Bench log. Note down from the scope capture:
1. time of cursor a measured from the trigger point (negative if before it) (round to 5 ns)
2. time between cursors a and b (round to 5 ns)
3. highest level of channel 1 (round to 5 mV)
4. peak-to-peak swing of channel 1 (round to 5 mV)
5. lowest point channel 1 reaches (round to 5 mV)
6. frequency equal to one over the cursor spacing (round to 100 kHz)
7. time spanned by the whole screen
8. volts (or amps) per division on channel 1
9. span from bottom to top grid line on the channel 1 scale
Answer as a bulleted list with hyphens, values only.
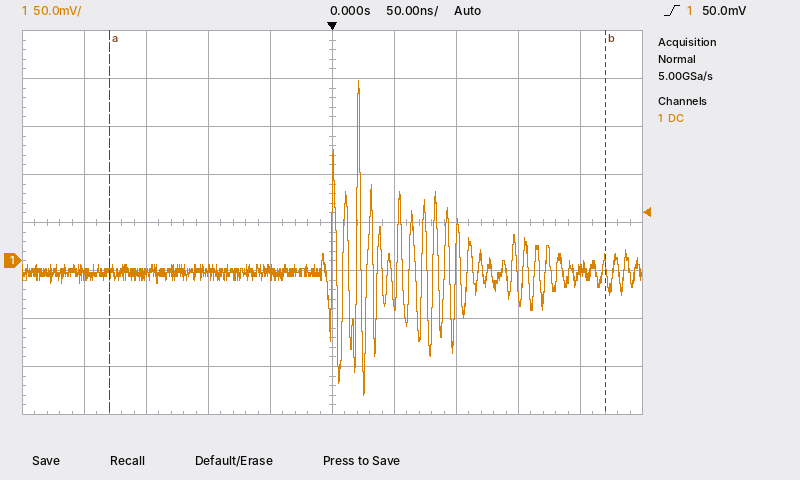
- -180 ns
- 400 ns
- 190 mV
- 330 mV
- -140 mV
- 2.5 MHz
- 500 ns
- 50 mV
- 400 mV
